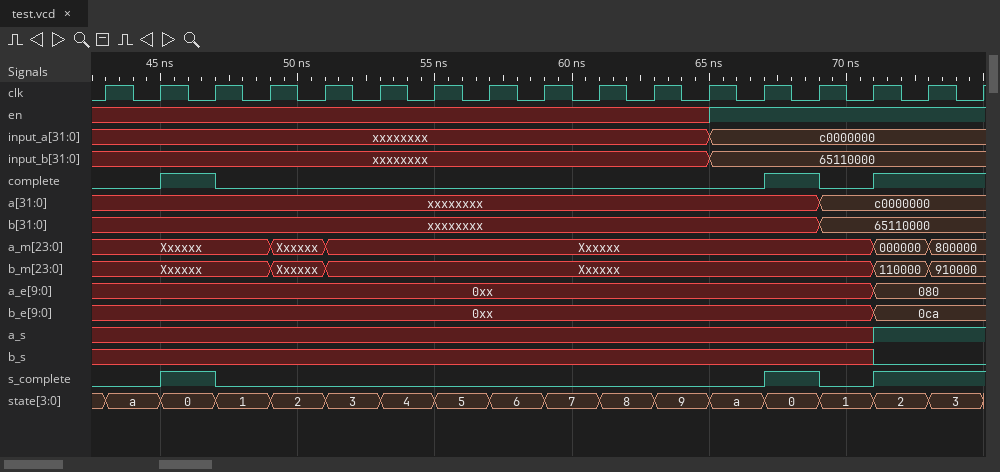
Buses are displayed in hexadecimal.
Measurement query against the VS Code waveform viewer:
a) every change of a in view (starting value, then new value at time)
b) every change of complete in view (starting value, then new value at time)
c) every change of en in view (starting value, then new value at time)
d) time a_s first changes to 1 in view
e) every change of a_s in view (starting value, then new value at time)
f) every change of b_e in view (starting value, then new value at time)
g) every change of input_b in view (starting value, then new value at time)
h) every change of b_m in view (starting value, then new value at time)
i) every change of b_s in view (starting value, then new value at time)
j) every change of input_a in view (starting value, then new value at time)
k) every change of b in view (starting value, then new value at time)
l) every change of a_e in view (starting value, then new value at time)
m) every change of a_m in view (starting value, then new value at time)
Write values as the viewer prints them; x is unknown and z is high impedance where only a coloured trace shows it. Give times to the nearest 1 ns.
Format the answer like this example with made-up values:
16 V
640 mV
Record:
xxxxxxxx, c0000000 at 69 ns
0, 1 at 45 ns, 0 at 47 ns, 1 at 67 ns, 0 at 69 ns, 1 at 71 ns
x, 1 at 65 ns
71 ns
x, 1 at 71 ns
0xx, 0ca at 71 ns
xxxxxxxx, 65110000 at 65 ns
Xxxxxx, Xxxxxx at 49 ns, Xxxxxx at 51 ns, 110000 at 71 ns, 910000 at 73 ns
x, 0 at 71 ns
xxxxxxxx, c0000000 at 65 ns
xxxxxxxx, 65110000 at 69 ns
0xx, 080 at 71 ns
Xxxxxx, Xxxxxx at 49 ns, Xxxxxx at 51 ns, 000000 at 71 ns, 800000 at 73 ns
